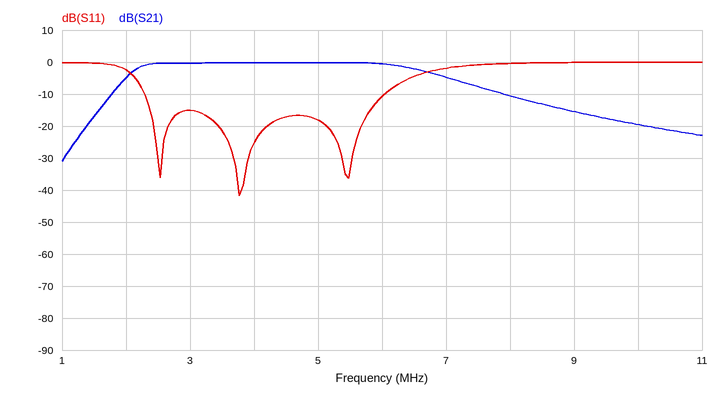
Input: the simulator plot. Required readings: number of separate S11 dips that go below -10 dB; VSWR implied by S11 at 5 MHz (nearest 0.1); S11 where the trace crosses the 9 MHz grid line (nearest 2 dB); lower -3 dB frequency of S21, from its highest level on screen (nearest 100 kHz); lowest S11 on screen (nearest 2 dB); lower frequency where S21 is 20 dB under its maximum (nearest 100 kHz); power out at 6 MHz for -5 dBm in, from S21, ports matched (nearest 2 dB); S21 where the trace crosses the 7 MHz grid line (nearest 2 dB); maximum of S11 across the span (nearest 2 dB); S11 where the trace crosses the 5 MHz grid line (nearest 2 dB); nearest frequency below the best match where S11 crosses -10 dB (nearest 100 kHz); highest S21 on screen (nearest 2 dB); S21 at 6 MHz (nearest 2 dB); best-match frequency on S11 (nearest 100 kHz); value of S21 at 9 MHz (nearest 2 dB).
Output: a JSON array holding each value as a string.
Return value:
["3", "1.3", "0 dB", "2.1 MHz", "-42 dB", "1.4 MHz", "-6 dBm", "-4 dB", "0 dB", "-18 dB", "2.3 MHz", "0 dB", "0 dB", "3.8 MHz", "-16 dB"]
